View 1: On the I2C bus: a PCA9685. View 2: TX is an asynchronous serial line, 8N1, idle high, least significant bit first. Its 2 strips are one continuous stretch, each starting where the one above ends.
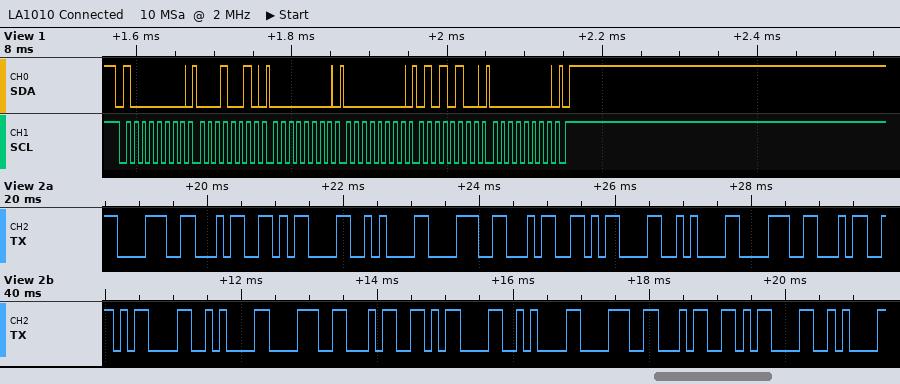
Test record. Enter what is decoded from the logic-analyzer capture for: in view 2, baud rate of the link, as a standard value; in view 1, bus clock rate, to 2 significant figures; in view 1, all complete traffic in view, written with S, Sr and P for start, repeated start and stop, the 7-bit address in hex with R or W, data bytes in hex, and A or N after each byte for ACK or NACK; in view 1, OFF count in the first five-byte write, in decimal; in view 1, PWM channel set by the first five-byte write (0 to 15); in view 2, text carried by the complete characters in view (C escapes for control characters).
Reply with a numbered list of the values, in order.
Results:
1. 9600 baud
2. 100 kHz
3. S 40W A 12 A 00 A 00 A 54 A 00 A P
4. 84
5. 3
6. "84\r\n84\r\n84\r\n84\r\n84\r\n"
